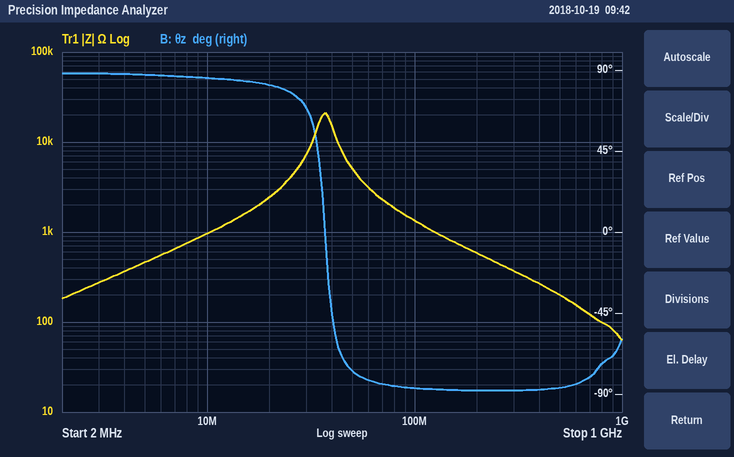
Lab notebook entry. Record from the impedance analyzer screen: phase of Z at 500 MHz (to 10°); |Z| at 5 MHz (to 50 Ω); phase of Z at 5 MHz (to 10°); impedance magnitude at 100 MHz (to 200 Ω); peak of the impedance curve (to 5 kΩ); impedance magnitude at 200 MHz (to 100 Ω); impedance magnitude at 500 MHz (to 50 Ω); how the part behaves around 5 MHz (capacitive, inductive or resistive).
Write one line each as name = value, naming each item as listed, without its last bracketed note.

phase of Z at 500 MHz = -90°
|Z| at 5 MHz = 450 Ω
phase of Z at 5 MHz = 90°
impedance magnitude at 100 MHz = 1.4 kΩ
peak of the impedance curve = 20 kΩ
impedance magnitude at 200 MHz = 600 Ω
impedance magnitude at 500 MHz = 200 Ω
how the part behaves around 5 MHz = inductive
